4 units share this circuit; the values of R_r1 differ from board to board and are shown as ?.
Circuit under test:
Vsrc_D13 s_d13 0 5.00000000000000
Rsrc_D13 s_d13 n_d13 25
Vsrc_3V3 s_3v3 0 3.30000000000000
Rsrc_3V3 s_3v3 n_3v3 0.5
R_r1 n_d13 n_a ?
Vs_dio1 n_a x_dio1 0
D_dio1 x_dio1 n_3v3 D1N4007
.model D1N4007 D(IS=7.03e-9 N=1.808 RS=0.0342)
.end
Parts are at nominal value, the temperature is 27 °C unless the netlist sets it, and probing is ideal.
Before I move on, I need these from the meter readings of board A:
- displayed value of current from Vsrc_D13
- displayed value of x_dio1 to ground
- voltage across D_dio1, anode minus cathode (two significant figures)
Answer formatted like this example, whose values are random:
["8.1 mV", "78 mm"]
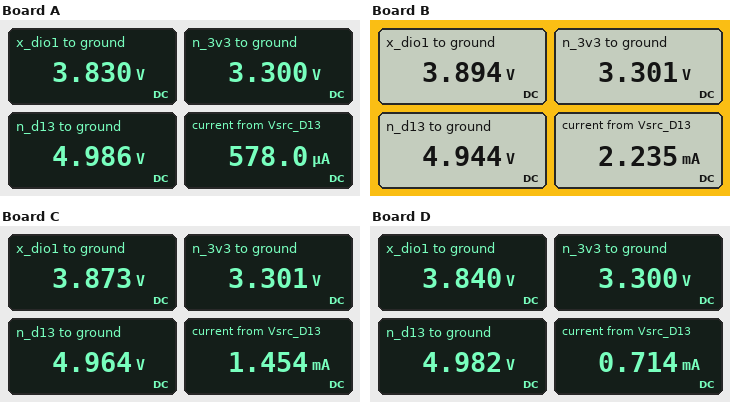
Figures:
["578.0 µA", "3.830 V", "530 mV"]
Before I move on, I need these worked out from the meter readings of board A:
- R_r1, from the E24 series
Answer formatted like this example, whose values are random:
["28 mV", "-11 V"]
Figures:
["2 kΩ"]
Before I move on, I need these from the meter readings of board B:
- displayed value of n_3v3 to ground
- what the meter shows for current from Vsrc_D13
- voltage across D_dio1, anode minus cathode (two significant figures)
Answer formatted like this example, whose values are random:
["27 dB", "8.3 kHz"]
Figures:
["3.301 V", "2.235 mA", "590 mV"]
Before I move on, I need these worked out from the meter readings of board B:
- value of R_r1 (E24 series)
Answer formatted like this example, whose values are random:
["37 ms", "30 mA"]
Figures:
["470 Ω"]
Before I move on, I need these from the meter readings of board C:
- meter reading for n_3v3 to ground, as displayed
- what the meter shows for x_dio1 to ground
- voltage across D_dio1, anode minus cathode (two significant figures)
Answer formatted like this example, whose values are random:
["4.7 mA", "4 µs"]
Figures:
["3.301 V", "3.873 V", "570 mV"]
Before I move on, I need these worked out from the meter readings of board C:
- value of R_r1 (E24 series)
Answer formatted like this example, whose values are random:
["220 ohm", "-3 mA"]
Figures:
["750 Ω"]
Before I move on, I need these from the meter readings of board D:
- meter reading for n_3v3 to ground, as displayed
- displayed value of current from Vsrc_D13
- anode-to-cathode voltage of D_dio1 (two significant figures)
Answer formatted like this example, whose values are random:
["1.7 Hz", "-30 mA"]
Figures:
["3.300 V", "0.714 mA", "540 mV"]
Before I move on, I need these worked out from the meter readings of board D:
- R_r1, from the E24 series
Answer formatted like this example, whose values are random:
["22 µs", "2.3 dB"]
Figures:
["1.6 kΩ"]
